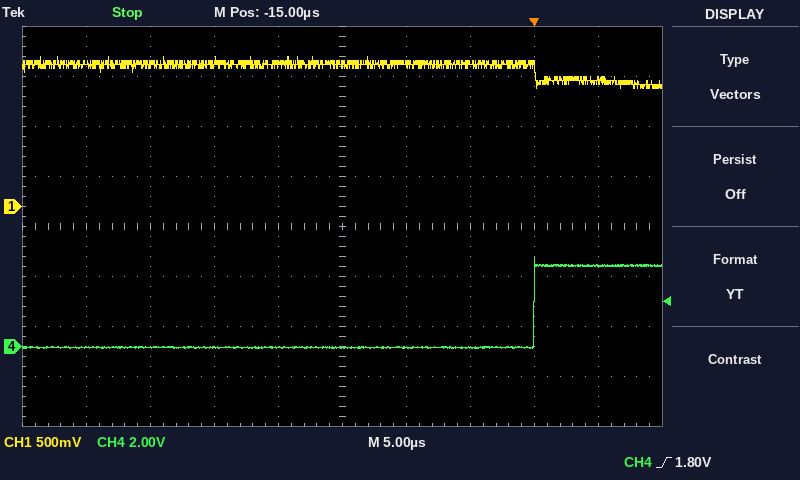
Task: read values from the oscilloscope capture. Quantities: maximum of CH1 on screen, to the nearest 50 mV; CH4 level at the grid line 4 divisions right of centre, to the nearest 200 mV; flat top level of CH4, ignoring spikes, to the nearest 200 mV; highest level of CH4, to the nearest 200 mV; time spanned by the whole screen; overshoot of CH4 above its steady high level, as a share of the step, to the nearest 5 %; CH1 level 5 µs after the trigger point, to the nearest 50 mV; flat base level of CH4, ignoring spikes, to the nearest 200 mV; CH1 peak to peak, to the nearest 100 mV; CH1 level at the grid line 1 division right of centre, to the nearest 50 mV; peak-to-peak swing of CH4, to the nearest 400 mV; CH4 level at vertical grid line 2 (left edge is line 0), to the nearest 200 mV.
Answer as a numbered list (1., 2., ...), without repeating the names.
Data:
1. 1.50 V
2. 3.2 V
3. 3.2 V
4. 3.6 V
5. 50 µs
6. 10 %
7. 1.25 V
8. 0.0 V
9. 300 mV
10. 1.40 V
11. 3.6 V
12. 0.0 V
